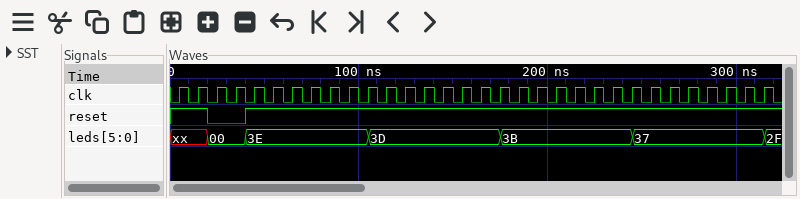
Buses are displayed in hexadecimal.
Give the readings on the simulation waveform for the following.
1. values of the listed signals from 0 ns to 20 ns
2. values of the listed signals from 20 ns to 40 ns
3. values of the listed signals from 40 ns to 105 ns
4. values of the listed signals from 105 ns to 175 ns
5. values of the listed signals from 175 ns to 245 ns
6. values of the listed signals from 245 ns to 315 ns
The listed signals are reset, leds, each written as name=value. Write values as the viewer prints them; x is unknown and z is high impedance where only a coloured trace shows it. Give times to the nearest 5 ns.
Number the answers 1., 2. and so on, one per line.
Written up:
1. reset=1, leds=xx
2. reset=0, leds=00
3. reset=1, leds=3E
4. reset=1, leds=3D
5. reset=1, leds=3B
6. reset=1, leds=37
